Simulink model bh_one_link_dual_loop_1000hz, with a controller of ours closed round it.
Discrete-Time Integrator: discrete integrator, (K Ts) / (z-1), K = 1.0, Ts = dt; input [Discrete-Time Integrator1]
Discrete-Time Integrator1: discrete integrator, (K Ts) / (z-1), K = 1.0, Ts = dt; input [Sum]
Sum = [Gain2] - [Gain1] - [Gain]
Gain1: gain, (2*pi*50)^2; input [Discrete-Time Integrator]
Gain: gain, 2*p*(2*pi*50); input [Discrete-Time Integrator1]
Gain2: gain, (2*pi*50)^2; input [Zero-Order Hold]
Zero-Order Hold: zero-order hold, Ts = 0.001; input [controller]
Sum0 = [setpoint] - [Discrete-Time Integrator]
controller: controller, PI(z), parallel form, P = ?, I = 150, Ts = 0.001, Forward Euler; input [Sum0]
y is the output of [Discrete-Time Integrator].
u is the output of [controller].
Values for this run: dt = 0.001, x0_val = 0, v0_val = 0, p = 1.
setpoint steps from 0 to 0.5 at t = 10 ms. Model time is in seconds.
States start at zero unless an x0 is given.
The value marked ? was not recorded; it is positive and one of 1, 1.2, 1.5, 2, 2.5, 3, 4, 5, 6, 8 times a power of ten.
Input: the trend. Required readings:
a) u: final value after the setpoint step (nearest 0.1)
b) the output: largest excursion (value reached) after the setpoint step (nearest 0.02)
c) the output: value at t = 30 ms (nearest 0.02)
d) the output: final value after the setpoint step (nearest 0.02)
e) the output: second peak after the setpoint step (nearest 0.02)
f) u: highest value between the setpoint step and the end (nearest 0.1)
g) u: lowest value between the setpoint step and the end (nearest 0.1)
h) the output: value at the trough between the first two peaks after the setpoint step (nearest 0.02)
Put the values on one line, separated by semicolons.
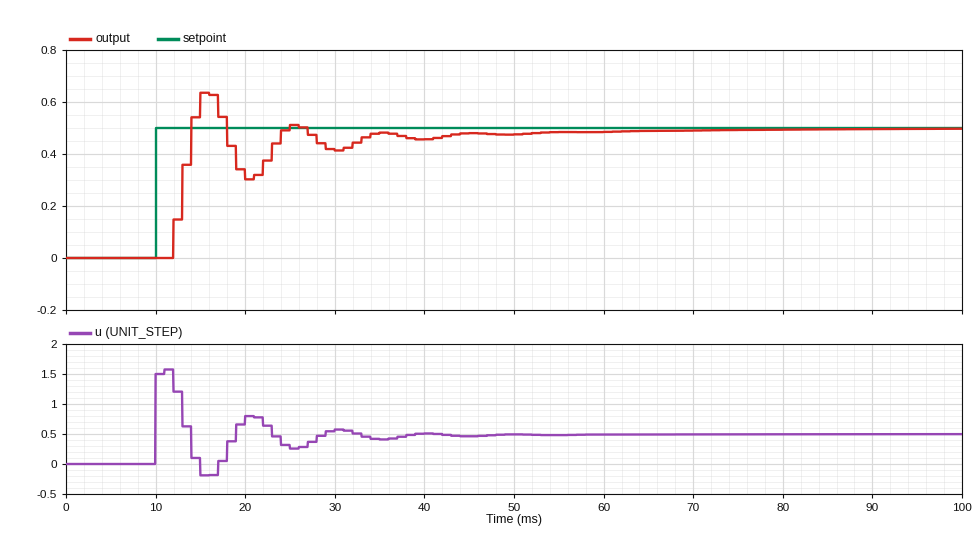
0.5; 0.64; 0.42; 0.50; 0.52; 1.6; -0.2; 0.30
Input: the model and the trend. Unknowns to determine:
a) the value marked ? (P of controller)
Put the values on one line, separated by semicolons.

3
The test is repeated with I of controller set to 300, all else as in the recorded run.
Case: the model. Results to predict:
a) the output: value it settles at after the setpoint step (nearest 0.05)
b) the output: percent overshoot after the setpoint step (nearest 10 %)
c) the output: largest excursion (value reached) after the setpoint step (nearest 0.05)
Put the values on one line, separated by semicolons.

0.50; 40 %; 0.70
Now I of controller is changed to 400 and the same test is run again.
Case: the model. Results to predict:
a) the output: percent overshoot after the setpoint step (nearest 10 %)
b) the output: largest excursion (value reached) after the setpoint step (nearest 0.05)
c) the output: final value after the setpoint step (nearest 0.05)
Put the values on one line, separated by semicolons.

50 %; 0.75; 0.50
